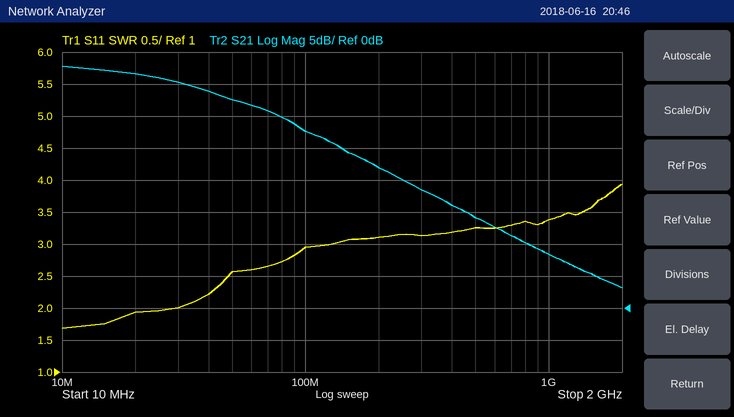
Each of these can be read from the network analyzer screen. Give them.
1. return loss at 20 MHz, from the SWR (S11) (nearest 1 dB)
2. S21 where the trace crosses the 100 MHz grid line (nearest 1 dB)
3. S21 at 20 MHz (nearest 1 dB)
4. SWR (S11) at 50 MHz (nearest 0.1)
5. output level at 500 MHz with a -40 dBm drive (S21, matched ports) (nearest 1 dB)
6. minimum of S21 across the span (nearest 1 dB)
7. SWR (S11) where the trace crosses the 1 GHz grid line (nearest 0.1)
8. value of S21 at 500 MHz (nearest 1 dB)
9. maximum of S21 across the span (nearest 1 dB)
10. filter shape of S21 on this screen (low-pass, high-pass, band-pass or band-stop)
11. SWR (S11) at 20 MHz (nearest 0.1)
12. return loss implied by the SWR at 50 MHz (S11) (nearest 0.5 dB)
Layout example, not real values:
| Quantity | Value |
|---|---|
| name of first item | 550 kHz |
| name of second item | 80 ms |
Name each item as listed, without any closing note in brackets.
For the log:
| Quantity | Value |
|---|---|
| return loss at 20 MHz, from the SWR (S11) | 10 dB |
| S21 where the trace crosses the 100 MHz grid line | 28 dB |
| S21 at 20 MHz | 37 dB |
| SWR (S11) at 50 MHz | 2.6 |
| output level at 500 MHz with a -40 dBm drive (S21, matched ports) | -26 dBm |
| minimum of S21 across the span | 3 dB |
| SWR (S11) where the trace crosses the 1 GHz grid line | 3.4 |
| value of S21 at 500 MHz | 14 dB |
| maximum of S21 across the span | 38 dB |
| filter shape of S21 on this screen | low-pass |
| SWR (S11) at 20 MHz | 1.9 |
| return loss implied by the SWR at 50 MHz (S11) | 7.0 dB |
